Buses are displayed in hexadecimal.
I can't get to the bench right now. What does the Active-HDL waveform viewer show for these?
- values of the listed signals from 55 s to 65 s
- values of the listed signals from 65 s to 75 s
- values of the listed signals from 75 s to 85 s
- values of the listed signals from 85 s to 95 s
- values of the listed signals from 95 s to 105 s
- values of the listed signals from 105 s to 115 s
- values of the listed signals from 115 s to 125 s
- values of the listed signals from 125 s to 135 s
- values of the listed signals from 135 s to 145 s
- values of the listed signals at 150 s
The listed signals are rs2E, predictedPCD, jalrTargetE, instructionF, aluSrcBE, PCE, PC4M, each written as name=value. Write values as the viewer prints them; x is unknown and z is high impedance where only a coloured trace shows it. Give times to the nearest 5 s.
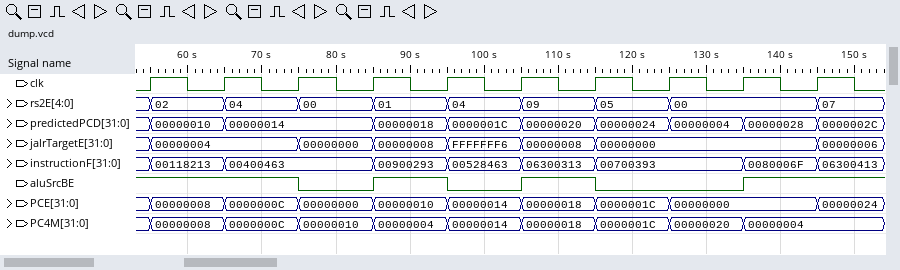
rs2E=02, predictedPCD=00000010, jalrTargetE=00000004, instructionF=00118213, aluSrcBE=1, PCE=00000008, PC4M=00000008
rs2E=04, predictedPCD=00000014, jalrTargetE=00000004, instructionF=00400463, aluSrcBE=1, PCE=0000000C, PC4M=0000000C
rs2E=00, predictedPCD=00000014, jalrTargetE=00000000, instructionF=00400463, aluSrcBE=0, PCE=00000000, PC4M=00000010
rs2E=01, predictedPCD=00000018, jalrTargetE=00000008, instructionF=00900293, aluSrcBE=1, PCE=00000010, PC4M=00000004
rs2E=04, predictedPCD=0000001C, jalrTargetE=FFFFFFF6, instructionF=00528463, aluSrcBE=0, PCE=00000014, PC4M=00000014
rs2E=09, predictedPCD=00000020, jalrTargetE=00000008, instructionF=06300313, aluSrcBE=1, PCE=00000018, PC4M=00000018
rs2E=05, predictedPCD=00000024, jalrTargetE=00000000, instructionF=00700393, aluSrcBE=0, PCE=0000001C, PC4M=0000001C
rs2E=00, predictedPCD=00000004, jalrTargetE=00000000, instructionF=00700393, aluSrcBE=0, PCE=00000000, PC4M=00000020
rs2E=00, predictedPCD=00000028, jalrTargetE=00000000, instructionF=0080006F, aluSrcBE=1, PCE=00000000, PC4M=00000004
rs2E=07, predictedPCD=0000002C, jalrTargetE=00000006, instructionF=06300413, aluSrcBE=1, PCE=00000024, PC4M=00000004
